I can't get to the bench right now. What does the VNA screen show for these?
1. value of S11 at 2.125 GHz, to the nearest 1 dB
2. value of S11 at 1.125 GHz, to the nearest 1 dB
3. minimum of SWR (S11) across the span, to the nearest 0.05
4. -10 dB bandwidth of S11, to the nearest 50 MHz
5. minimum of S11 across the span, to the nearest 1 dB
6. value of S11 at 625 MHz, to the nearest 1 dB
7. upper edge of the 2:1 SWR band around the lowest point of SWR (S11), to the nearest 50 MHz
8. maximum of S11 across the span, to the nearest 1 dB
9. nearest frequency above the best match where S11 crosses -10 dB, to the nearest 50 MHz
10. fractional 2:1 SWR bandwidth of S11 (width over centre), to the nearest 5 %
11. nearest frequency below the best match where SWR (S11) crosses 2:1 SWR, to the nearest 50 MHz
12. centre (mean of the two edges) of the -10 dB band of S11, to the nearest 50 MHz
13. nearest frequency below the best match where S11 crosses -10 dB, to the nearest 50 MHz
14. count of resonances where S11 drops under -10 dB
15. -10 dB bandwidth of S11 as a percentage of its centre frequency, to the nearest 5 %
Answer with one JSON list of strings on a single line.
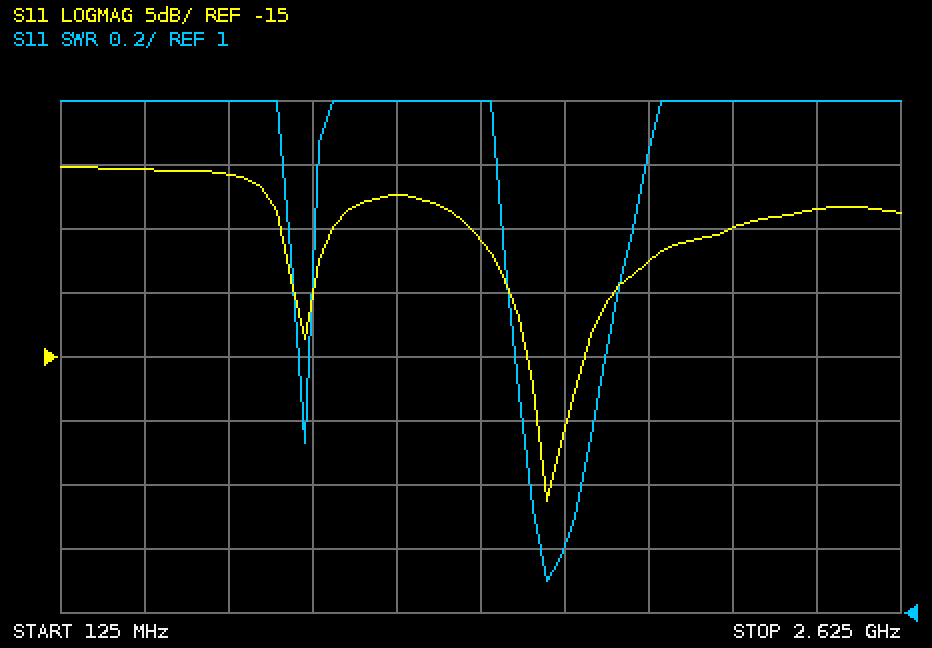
["-5 dB", "-2 dB", "1.10", "300 MHz", "-26 dB", "-1 dB", "1.80 GHz", "0 dB", "1.75 GHz", "20 %", "1.45 GHz", "1.60 GHz", "1.45 GHz", "2", "20 %"]
